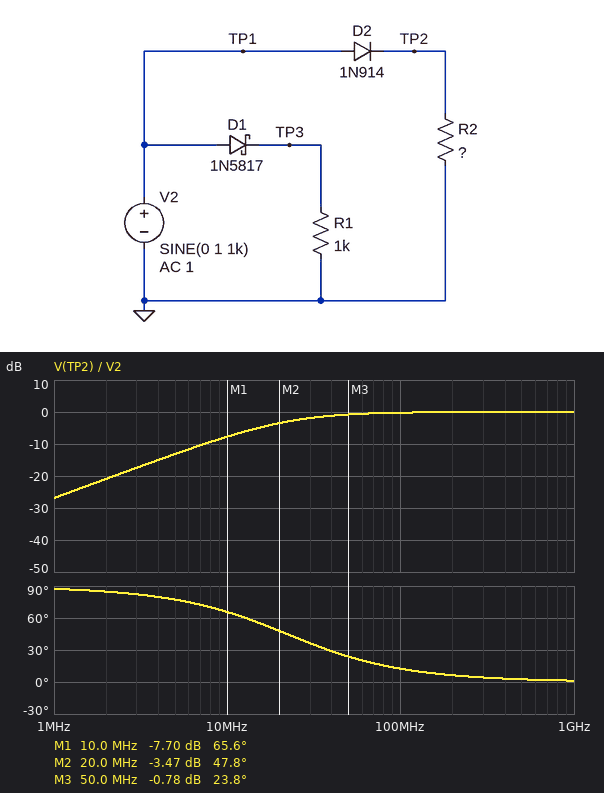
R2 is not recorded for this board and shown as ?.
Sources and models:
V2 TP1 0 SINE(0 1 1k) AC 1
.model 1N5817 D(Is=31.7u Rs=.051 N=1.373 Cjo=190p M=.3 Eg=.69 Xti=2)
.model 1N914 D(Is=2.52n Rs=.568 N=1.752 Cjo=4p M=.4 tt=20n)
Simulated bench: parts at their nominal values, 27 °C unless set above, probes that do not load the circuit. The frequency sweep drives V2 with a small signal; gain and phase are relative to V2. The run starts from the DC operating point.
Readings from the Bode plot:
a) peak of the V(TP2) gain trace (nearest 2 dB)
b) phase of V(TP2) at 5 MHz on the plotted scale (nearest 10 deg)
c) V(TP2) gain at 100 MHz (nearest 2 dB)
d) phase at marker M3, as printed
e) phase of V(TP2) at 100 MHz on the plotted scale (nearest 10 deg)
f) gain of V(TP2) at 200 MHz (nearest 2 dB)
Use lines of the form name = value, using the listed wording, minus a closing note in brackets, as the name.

peak of the V(TP2) gain trace = 0 dB
phase of V(TP2) at 5 MHz on the plotted scale = 80 deg
V(TP2) gain at 100 MHz = 0 dB
phase at marker M3, as printed = 23.8 deg
phase of V(TP2) at 100 MHz on the plotted scale = 10 deg
gain of V(TP2) at 200 MHz = 0 dB
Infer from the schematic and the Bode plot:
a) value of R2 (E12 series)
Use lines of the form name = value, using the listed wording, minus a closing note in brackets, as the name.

value of R2 = 1.8 kΩ
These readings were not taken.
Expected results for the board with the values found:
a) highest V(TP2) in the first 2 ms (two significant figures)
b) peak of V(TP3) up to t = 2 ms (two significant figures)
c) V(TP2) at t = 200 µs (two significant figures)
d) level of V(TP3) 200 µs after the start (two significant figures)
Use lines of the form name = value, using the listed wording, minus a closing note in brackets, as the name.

highest V(TP2) in the first 2 ms = 480 mV
peak of V(TP3) up to t = 2 ms = 880 mV
V(TP2) at t = 200 µs = 430 mV
level of V(TP3) 200 µs after the start = 830 mV
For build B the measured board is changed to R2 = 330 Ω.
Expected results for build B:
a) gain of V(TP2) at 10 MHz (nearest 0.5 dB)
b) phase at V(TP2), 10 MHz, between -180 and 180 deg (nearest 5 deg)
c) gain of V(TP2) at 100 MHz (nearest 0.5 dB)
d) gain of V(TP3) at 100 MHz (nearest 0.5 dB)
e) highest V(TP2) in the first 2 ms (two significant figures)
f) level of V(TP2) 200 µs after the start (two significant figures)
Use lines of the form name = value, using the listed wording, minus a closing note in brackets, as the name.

gain of V(TP2) at 10 MHz = -21.5 dB
phase at V(TP2), 10 MHz, between -180 and 180 deg = 85 deg
gain of V(TP2) at 100 MHz = -4.0 dB
gain of V(TP3) at 100 MHz = 0 dB
highest V(TP2) in the first 2 ms = 410 mV
level of V(TP2) 200 µs after the start = 360 mV
